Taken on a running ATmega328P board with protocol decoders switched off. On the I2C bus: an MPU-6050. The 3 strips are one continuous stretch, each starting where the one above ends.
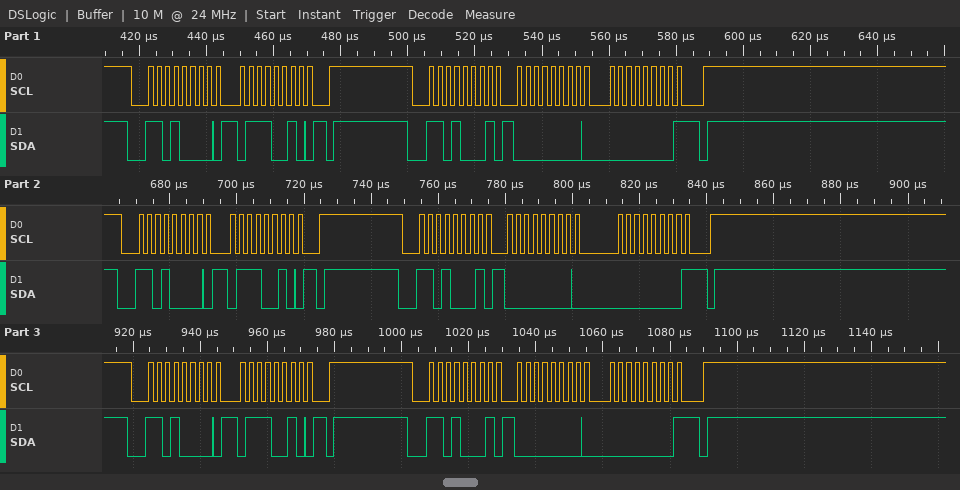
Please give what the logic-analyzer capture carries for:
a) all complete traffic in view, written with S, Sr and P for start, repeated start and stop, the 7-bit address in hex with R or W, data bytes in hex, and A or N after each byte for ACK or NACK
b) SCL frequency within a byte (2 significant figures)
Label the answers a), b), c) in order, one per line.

a) S 68W A 72 A P S 68R A 00 A 00 N P S 68W A 72 A P S 68R A 00 A 00 N P S 68W A 72 A P S 68R A 00 A 00 N P
b) 400 kHz
